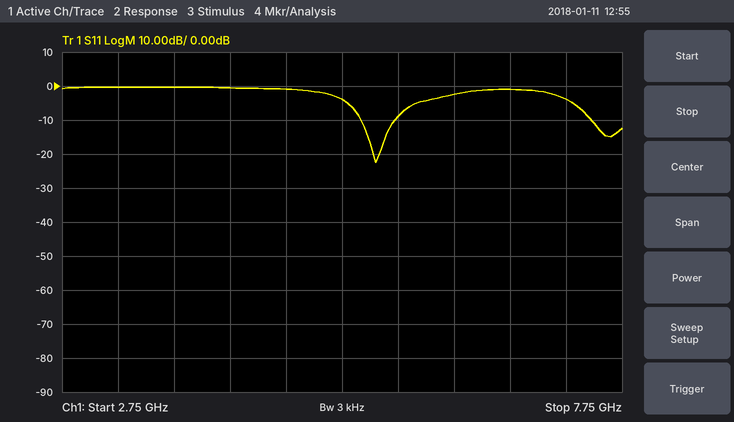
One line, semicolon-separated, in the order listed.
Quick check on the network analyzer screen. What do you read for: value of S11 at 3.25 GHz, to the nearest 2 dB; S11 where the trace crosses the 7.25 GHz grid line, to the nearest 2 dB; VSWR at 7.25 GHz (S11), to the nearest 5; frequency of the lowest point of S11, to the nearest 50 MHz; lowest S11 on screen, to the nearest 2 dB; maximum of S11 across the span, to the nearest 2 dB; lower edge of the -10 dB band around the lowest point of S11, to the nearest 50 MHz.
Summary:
0 dB; -4 dB; 5; 5.55 GHz; -22 dB; 0 dB; 5.40 GHz
